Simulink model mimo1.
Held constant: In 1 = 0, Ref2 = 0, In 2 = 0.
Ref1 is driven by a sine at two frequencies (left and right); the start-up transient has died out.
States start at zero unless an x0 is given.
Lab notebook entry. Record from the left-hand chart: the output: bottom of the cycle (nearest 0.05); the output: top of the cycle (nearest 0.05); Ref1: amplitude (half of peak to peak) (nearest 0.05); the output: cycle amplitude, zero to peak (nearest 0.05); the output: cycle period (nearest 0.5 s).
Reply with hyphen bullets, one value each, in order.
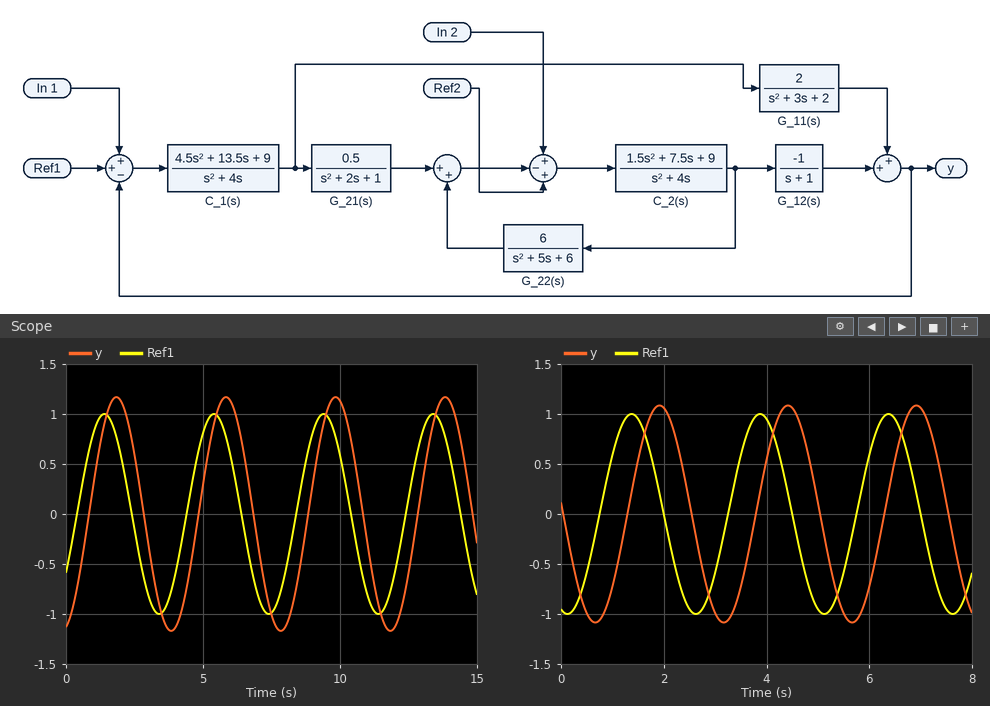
- -1.15
- 1.15
- 1.00
- 1.15
- 4.0 s
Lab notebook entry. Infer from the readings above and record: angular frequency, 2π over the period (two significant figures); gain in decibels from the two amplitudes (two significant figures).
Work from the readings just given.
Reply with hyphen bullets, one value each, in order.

- 1.6 rad/s
- 1.2 dB
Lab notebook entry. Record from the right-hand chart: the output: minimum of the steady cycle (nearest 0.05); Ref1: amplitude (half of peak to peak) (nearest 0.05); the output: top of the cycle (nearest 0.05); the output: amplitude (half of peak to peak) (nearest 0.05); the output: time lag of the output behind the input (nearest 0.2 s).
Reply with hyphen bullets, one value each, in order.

- -1.10
- 1.00
- 1.10
- 1.10
- 0.6 s
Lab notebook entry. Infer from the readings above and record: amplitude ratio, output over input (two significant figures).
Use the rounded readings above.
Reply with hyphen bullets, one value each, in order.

- 1.1
